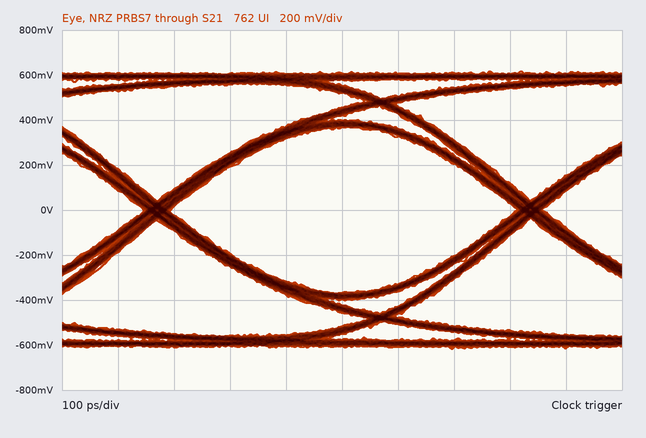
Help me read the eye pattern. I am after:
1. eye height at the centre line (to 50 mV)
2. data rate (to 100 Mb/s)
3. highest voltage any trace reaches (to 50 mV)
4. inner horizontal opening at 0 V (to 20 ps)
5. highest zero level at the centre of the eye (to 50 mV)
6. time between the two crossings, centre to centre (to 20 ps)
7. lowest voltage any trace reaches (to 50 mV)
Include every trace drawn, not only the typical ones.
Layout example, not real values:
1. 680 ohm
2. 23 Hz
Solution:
1. 750 mV
2. 1.5 Gb/s
3. 600 mV
4. 620 ps
5. -350 mV
6. 660 ps
7. -600 mV
